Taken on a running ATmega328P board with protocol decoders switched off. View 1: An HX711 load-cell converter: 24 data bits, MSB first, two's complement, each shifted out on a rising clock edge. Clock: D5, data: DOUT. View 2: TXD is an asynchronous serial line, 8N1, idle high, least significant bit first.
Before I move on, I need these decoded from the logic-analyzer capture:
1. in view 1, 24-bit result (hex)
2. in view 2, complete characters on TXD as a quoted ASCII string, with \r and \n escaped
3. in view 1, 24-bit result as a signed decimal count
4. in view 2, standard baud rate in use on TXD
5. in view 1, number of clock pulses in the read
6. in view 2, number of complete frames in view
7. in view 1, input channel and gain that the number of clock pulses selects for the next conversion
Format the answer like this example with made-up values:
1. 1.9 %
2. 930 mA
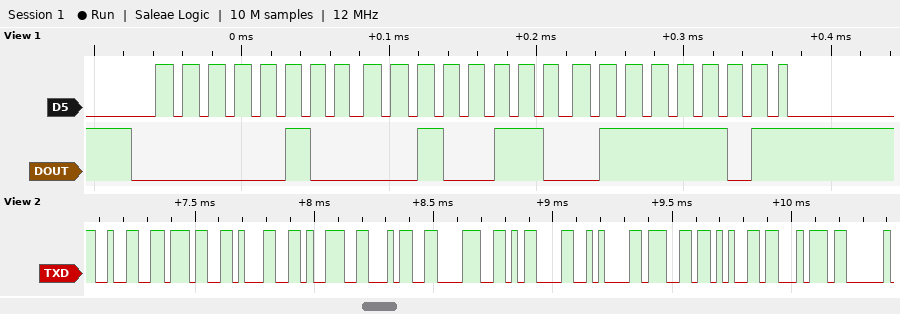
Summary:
1. 0x04267D
2. "271948\r\nget"
3. 271997
4. 38400 baud
5. 25
6. 11
7. channel A, gain 128
